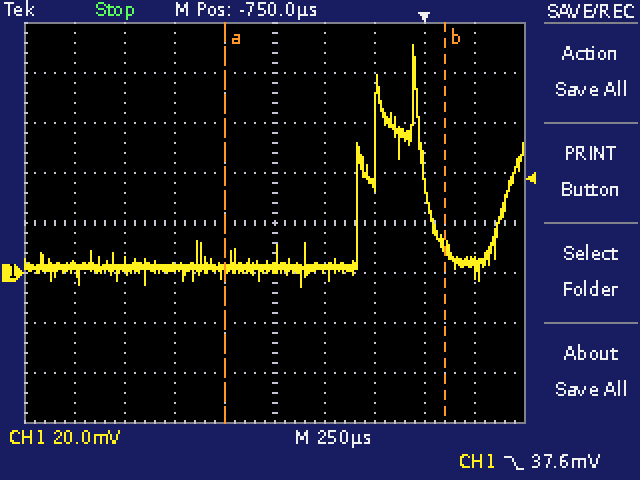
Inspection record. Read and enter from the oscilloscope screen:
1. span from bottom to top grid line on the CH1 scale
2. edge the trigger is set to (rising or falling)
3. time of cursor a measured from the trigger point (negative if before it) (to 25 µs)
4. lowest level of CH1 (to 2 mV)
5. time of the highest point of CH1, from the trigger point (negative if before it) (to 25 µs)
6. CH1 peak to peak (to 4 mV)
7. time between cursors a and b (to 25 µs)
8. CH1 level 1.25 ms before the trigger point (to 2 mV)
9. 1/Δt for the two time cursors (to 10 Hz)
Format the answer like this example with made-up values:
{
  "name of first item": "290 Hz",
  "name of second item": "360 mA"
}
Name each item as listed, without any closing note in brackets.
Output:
{
  "span from bottom to top grid line on the CH1 scale": "160 mV",
  "edge the trigger is set to": "falling",
  "time of cursor a measured from the trigger point (negative if before it)": "-1.000 ms",
  "lowest level of CH1": "-6 mV",
  "time of the highest point of CH1, from the trigger point (negative if before it)": "-50 µs",
  "CH1 peak to peak": "96 mV",
  "time between cursors a and b": "1.100 ms",
  "CH1 level 1.25 ms before the trigger point": "2 mV",
  "1/Δt for the two time cursors": "910 Hz"
}
